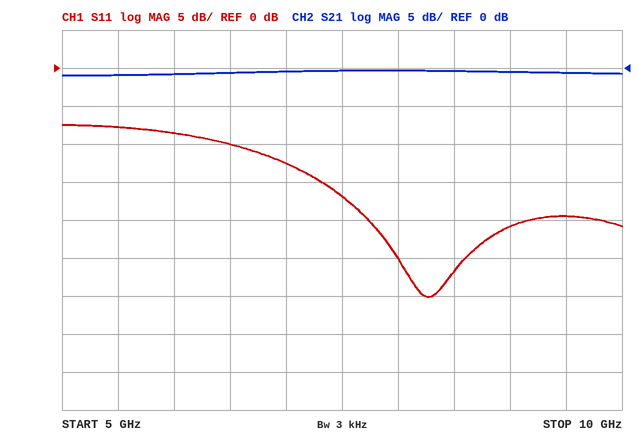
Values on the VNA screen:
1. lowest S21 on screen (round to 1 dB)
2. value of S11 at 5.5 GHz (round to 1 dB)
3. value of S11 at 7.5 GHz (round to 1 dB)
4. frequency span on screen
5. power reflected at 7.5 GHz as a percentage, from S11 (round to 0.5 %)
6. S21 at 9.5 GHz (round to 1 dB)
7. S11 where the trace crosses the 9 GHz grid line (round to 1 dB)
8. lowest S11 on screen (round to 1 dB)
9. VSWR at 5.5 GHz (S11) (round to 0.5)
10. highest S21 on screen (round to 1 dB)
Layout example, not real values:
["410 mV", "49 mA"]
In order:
["-1 dB", "-8 dB", "-17 dB", "5 GHz", "2.0 %", "-1 dB", "-21 dB", "-30 dB", "2.5", "0 dB"]
